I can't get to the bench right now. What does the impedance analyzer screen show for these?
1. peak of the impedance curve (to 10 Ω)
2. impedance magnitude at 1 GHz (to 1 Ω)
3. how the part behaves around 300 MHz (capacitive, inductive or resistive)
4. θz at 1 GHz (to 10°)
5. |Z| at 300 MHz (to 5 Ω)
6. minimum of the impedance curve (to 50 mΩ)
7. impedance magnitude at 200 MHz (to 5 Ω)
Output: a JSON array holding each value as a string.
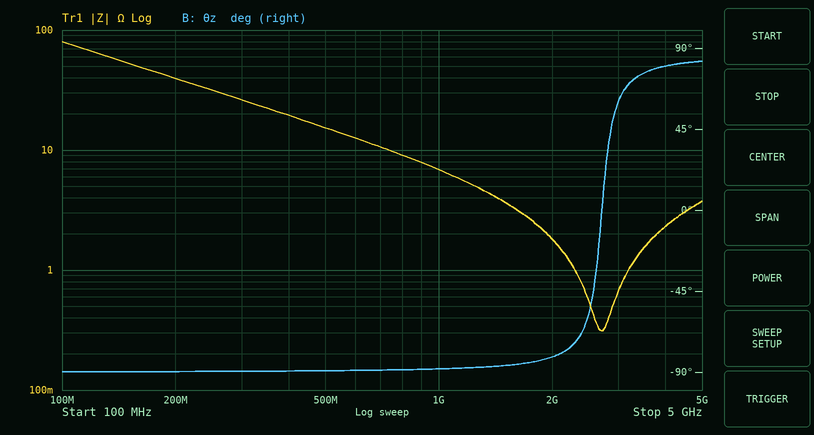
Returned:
["80 Ω", "7 Ω", "capacitive", "-90°", "25 Ω", "300 mΩ", "40 Ω"]
